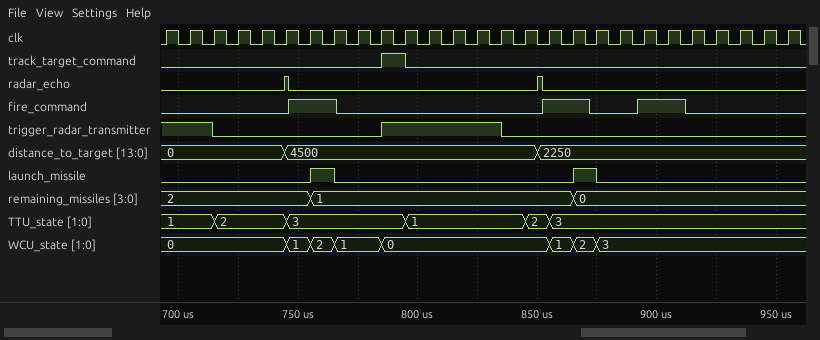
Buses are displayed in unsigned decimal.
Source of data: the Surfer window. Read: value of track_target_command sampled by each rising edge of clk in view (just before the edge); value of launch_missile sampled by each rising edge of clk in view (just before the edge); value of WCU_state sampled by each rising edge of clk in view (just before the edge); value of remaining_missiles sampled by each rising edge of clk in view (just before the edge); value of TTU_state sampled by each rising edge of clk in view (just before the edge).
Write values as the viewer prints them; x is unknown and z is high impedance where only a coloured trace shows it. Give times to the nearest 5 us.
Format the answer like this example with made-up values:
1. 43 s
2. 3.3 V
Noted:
1. 0 0 0 0 0 0 0 0 0 0 1 0 0 0 0 0 0 0 0 0 0 0 0 0 0 0 0
2. 0 0 0 0 0 0 0 1 0 0 0 0 0 0 0 0 0 0 1 0 0 0 0 0 0 0 0
3. 0, 0, 0, 0, 0, 0, 1, 2, 1, 1, 0, 0, 0, 0, 0, 0, 0, 1, 2, 3, 3, 3, 3, 3, 3, 3, 3
4. 2, 2, 2, 2, 2, 2, 2, 1, 1, 1, 1, 1, 1, 1, 1, 1, 1, 1, 0, 0, 0, 0, 0, 0, 0, 0, 0
5. 1, 1, 1, 2, 2, 2, 3, 3, 3, 3, 3, 1, 1, 1, 1, 1, 2, 3, 3, 3, 3, 3, 3, 3, 3, 3, 3
